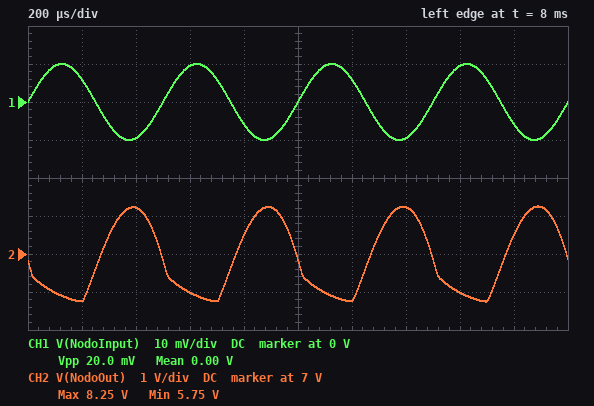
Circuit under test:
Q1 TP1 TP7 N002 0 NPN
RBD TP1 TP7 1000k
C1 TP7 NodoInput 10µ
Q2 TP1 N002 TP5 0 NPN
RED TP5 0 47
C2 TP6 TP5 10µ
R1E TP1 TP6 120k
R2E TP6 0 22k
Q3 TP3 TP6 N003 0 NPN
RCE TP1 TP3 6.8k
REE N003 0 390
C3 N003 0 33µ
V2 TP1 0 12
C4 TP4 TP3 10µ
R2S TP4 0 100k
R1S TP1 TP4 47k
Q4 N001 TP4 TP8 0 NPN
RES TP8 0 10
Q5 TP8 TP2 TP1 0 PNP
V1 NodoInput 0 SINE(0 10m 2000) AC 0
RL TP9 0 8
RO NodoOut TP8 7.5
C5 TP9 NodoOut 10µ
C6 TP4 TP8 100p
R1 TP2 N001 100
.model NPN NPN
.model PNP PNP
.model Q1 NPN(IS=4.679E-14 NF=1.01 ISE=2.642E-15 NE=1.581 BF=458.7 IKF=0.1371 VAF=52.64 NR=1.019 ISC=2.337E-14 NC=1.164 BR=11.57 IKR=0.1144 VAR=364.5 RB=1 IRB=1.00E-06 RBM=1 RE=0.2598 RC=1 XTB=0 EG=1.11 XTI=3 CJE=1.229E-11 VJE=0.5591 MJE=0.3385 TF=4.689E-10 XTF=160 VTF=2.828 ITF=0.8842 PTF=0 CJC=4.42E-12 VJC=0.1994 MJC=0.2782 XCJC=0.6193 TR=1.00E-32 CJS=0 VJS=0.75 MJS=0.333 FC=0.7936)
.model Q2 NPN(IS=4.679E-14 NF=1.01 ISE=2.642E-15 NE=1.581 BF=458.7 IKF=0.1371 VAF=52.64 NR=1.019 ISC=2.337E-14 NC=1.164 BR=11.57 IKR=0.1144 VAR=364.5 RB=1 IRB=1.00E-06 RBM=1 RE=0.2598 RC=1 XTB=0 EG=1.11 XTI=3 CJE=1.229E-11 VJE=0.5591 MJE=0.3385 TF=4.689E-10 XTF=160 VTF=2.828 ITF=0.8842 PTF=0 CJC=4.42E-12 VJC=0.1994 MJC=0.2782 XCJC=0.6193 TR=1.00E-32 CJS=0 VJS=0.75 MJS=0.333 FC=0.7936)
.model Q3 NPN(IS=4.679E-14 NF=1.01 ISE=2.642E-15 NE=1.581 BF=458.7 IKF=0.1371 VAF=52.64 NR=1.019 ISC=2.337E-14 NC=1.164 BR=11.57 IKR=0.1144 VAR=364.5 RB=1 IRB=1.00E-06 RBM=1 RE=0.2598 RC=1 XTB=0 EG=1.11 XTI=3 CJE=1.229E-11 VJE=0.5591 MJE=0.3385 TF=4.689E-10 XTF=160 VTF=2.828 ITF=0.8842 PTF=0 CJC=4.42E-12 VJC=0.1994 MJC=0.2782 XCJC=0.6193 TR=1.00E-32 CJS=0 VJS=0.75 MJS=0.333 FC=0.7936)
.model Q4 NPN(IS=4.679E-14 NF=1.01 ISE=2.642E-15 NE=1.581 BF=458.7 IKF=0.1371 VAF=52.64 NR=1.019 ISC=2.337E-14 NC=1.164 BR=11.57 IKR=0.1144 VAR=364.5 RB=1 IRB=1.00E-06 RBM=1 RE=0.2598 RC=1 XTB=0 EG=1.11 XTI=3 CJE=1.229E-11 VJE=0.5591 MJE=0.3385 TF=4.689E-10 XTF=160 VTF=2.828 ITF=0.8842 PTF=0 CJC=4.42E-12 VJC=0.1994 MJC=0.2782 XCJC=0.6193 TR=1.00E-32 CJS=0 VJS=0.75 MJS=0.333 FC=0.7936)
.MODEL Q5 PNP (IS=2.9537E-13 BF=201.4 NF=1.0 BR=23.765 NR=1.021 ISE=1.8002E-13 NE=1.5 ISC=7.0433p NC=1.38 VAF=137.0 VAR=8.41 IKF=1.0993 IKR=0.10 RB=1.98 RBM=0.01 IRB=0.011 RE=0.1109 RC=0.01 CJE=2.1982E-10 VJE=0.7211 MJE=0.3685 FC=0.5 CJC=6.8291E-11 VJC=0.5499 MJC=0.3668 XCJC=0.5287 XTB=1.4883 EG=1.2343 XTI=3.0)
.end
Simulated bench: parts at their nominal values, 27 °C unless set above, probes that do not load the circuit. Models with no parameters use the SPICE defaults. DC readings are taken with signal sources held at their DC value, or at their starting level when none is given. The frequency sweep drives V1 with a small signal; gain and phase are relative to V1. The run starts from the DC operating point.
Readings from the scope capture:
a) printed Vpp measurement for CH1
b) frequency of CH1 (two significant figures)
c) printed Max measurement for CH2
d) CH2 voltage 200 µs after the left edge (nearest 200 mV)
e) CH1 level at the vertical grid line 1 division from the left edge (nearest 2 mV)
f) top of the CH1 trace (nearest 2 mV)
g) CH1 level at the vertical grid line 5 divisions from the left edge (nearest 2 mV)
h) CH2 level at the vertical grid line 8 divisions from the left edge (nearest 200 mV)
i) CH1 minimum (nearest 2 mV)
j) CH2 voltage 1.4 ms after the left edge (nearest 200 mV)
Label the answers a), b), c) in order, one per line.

a) 20.0 mV
b) 2.0 kHz
c) 8.25 V
d) 5.8 V
e) 6 mV
f) 10 mV
g) 0 V
h) 6.0 V
i) -10 mV
j) 8.2 V
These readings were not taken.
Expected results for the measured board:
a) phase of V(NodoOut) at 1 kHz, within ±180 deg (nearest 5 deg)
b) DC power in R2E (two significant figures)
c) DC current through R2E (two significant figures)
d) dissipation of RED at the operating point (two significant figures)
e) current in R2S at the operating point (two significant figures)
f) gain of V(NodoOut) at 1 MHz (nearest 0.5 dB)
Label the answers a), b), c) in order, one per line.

a) -170 deg
b) 94 µW
c) 65 µA
d) 240 mW
e) 64 µA
f) 33.5 dB
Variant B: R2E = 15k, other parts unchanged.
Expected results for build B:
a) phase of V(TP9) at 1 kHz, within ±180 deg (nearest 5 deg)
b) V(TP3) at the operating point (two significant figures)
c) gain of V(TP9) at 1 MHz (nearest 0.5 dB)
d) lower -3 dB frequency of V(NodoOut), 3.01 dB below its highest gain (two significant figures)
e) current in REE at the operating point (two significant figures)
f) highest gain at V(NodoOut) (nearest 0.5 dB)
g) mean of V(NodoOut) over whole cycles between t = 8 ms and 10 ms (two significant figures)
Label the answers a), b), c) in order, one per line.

a) -125 deg
b) 4.8 V
c) 40.5 dB
d) 160 Hz
e) 1.1 mA
f) 45.0 dB
g) 5.6 V
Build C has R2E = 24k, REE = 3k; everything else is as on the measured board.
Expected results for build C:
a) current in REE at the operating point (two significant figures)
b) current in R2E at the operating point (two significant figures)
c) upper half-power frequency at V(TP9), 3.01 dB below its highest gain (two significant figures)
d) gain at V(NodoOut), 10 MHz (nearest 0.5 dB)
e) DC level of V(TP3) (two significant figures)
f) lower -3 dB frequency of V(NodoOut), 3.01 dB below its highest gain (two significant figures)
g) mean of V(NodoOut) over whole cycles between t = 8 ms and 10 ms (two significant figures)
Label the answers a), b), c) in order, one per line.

a) 390 µA
b) 80 µA
c) 41 MHz
d) 31.5 dB
e) 9.4 V
f) 68 Hz
g) 5.6 V
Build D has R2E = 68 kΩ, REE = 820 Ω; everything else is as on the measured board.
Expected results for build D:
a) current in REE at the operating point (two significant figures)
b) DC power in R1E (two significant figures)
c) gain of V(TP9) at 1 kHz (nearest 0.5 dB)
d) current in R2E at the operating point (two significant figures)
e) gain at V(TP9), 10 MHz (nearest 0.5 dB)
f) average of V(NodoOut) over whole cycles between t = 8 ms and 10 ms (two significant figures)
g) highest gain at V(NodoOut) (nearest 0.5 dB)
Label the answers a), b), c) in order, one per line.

a) 1.6 mA
b) 820 µW
c) 15.5 dB
d) 31 µA
e) 20.0 dB
f) 6.6 V
g) 22.5 dB
